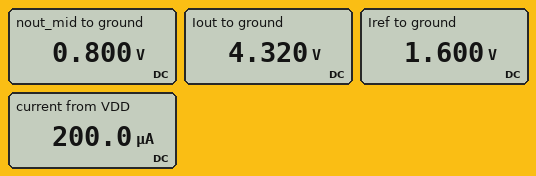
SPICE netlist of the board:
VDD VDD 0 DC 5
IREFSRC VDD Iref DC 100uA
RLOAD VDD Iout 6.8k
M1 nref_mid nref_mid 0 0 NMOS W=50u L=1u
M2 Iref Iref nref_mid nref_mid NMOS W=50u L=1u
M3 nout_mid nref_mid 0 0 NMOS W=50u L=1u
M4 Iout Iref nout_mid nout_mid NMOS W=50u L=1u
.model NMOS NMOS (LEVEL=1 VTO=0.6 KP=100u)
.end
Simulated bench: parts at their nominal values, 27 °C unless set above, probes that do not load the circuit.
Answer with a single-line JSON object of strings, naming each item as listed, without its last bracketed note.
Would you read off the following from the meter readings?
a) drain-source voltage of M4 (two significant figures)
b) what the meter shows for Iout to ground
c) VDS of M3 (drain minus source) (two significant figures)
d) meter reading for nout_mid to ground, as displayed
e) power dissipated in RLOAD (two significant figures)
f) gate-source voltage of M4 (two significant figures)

{"drain-source voltage of M4": "3.5 V", "what the meter shows for Iout to ground": "4.320 V", "VDS of M3 (drain minus source)": "800 mV", "meter reading for nout_mid to ground, as displayed": "0.800 V", "power dissipated in RLOAD": "68 µW", "gate-source voltage of M4": "800 mV"}
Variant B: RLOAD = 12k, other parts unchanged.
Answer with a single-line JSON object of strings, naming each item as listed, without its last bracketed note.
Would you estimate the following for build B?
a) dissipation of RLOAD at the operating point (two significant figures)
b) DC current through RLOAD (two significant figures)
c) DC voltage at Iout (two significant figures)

{"dissipation of RLOAD at the operating point": "120 µW", "DC current through RLOAD": "100 µA", "DC voltage at Iout": "3.8 V"}
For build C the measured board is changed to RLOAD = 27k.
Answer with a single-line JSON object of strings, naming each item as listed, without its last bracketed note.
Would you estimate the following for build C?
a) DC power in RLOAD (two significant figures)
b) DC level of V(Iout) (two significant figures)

{"DC power in RLOAD": "270 µW", "DC level of V(Iout)": "2.3 V"}
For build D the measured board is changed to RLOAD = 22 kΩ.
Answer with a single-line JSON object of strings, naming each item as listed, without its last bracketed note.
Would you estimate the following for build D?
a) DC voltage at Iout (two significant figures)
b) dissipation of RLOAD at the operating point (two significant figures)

{"DC voltage at Iout": "2.8 V", "dissipation of RLOAD at the operating point": "220 µW"}
